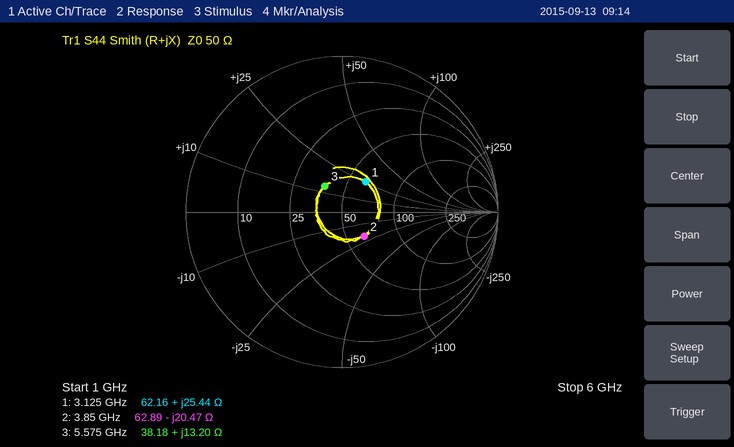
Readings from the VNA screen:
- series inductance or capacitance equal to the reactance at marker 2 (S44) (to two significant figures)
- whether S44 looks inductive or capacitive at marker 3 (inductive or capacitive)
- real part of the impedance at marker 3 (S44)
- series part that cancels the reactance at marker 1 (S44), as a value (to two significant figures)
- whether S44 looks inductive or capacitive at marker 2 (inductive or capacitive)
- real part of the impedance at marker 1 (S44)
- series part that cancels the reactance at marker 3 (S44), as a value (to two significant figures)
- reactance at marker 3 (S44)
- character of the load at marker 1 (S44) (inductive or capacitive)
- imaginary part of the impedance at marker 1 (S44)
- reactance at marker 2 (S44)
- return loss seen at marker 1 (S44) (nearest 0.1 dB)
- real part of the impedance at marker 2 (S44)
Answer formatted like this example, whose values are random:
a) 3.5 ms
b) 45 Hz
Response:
a) 2.0 pF
b) inductive
c) 38.18 Ω
d) 2.0 pF
e) capacitive
f) 62.16 Ω
g) 2.2 pF
h) +13.20 Ω
i) inductive
j) +25.44 Ω
k) -20.47 Ω
l) 12.2 dB
m) 62.89 Ω
